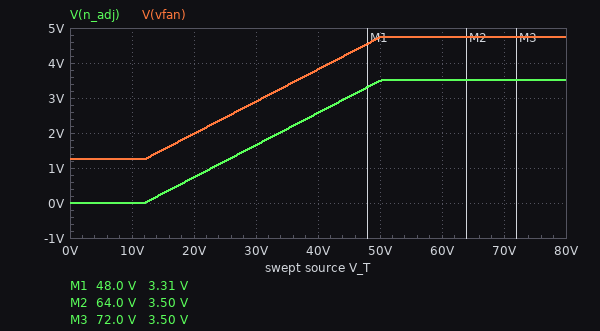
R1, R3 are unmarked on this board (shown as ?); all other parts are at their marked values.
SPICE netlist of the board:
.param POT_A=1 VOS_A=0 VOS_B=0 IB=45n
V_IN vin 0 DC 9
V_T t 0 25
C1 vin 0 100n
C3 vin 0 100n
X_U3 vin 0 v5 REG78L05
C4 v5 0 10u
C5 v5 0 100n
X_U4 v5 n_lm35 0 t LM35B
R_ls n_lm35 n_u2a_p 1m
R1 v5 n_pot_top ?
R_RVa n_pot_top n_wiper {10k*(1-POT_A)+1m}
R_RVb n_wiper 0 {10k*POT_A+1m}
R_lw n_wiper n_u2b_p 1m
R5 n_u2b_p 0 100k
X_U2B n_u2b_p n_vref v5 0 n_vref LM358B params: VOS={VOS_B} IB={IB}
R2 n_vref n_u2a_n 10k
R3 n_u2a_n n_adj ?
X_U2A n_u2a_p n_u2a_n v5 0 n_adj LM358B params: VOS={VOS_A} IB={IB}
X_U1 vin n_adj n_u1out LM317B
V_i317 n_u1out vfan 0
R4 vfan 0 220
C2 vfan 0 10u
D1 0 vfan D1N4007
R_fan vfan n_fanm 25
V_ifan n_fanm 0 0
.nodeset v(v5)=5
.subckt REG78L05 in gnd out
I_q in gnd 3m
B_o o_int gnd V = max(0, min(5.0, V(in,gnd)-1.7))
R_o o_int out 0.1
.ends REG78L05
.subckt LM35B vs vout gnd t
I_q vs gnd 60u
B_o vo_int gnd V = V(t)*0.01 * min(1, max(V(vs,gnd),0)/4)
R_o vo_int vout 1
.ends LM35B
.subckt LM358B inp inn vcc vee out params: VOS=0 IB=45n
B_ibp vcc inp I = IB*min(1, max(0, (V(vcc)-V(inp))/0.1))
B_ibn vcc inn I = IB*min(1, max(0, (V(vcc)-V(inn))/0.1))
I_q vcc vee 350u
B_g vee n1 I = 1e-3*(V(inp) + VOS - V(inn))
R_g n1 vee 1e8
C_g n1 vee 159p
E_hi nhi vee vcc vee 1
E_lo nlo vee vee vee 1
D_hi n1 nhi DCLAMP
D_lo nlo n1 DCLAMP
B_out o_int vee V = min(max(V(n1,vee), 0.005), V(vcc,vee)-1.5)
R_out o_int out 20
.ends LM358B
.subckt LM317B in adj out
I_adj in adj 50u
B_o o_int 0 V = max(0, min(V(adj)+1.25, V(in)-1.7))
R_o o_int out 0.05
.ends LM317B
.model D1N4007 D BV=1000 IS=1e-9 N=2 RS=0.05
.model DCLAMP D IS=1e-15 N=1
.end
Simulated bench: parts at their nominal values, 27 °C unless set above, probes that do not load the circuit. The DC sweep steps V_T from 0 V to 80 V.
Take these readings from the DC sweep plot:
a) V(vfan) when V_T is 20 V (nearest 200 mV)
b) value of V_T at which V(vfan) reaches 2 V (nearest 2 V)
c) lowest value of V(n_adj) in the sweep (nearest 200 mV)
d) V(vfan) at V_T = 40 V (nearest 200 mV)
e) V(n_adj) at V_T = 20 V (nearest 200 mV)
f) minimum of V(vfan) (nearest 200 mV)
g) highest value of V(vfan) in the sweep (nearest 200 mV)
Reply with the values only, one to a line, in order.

2.0 V
20 V
0 V
3.8 V
800 mV
1.2 V
4.8 V
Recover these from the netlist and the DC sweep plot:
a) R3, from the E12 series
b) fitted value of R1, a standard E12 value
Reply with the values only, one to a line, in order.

82 kΩ
330 kΩ
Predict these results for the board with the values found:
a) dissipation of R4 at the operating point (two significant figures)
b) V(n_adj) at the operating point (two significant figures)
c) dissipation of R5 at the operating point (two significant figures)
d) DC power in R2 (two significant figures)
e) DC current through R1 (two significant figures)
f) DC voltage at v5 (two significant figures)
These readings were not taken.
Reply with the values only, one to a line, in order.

27 mW
1.2 V
180 nW
1.3 µW
15 µA
5.0 V
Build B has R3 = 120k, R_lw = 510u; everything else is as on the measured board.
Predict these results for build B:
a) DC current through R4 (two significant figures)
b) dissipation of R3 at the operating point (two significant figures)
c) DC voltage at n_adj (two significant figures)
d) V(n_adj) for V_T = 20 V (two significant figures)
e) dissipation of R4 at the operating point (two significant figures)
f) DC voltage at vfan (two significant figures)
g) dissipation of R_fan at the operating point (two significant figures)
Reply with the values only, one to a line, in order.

13 mA
16 µW
1.6 V
980 mV
38 mW
2.9 V
330 mW
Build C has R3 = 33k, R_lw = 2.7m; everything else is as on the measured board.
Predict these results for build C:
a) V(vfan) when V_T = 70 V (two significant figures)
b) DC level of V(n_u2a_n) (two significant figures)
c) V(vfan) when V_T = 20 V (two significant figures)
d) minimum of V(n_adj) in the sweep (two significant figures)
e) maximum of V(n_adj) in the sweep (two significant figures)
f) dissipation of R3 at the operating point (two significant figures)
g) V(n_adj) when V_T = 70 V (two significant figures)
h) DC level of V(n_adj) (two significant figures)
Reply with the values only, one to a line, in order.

3.8 V
250 mV
1.7 V
6.1 mV
3.0 V
4.4 µW
2.6 V
630 mV
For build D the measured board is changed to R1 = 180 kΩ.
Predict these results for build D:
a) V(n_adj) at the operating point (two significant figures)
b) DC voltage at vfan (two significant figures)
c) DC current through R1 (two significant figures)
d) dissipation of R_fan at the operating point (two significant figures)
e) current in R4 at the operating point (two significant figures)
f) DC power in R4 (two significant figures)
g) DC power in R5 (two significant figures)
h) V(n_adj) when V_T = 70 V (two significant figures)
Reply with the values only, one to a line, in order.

320 mV
1.6 V
26 µA
98 mW
7.1 mA
11 mW
580 nW
3.5 V
